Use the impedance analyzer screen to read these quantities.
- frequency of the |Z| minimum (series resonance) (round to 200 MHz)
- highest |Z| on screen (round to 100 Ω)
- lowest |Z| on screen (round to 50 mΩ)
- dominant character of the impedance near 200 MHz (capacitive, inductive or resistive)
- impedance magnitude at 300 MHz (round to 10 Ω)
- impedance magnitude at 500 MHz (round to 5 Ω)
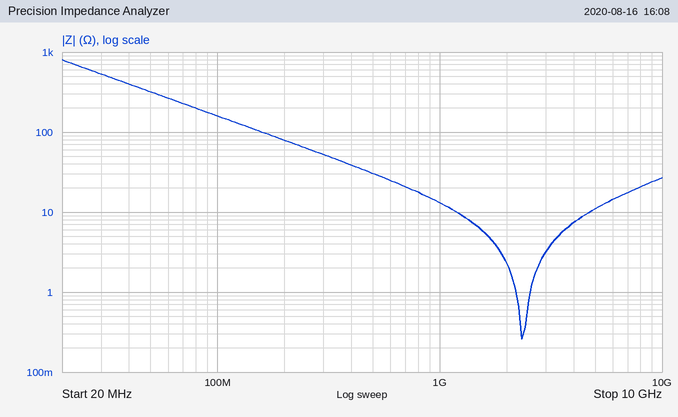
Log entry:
2.4 GHz
800 Ω
250 mΩ
capacitive
50 Ω
30 Ω
